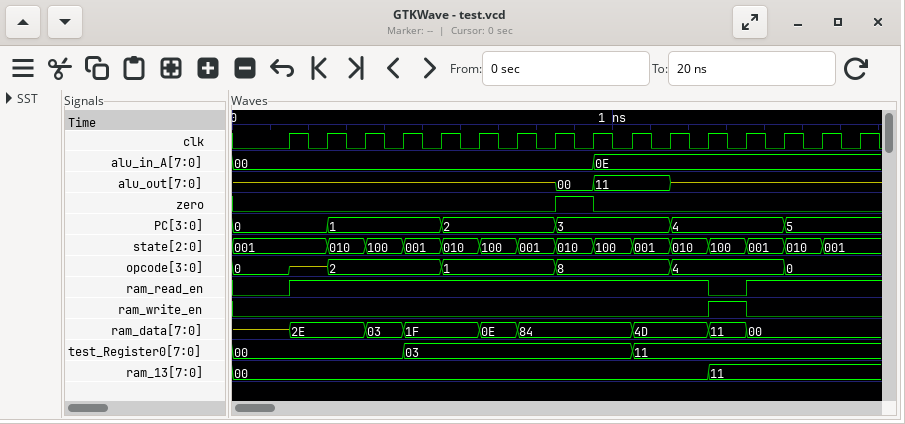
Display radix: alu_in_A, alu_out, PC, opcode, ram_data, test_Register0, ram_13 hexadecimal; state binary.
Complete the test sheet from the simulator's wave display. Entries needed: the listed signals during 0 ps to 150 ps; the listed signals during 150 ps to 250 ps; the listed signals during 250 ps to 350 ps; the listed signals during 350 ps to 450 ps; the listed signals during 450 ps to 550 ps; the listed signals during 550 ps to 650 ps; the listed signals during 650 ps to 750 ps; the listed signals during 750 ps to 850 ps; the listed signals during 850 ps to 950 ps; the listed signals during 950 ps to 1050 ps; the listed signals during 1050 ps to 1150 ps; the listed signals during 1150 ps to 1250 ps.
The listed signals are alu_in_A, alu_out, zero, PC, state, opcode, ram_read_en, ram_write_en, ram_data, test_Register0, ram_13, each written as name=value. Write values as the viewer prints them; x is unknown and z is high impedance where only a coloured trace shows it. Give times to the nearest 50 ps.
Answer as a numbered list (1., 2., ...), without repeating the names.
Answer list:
1. alu_in_A=00, alu_out=z, zero=0, PC=0, state=001, opcode=0, ram_read_en=0, ram_write_en=0, ram_data=z, test_Register0=00, ram_13=00
2. alu_in_A=00, alu_out=z, zero=0, PC=0, state=001, opcode=z, ram_read_en=1, ram_write_en=0, ram_data=2E, test_Register0=00, ram_13=00
3. alu_in_A=00, alu_out=z, zero=0, PC=1, state=010, opcode=2, ram_read_en=1, ram_write_en=0, ram_data=2E, test_Register0=00, ram_13=00
4. alu_in_A=00, alu_out=z, zero=0, PC=1, state=100, opcode=2, ram_read_en=1, ram_write_en=0, ram_data=03, test_Register0=00, ram_13=00
5. alu_in_A=00, alu_out=z, zero=0, PC=1, state=001, opcode=2, ram_read_en=1, ram_write_en=0, ram_data=1F, test_Register0=03, ram_13=00
6. alu_in_A=00, alu_out=z, zero=0, PC=2, state=010, opcode=1, ram_read_en=1, ram_write_en=0, ram_data=1F, test_Register0=03, ram_13=00
7. alu_in_A=00, alu_out=z, zero=0, PC=2, state=100, opcode=1, ram_read_en=1, ram_write_en=0, ram_data=0E, test_Register0=03, ram_13=00
8. alu_in_A=00, alu_out=z, zero=0, PC=2, state=001, opcode=1, ram_read_en=1, ram_write_en=0, ram_data=84, test_Register0=03, ram_13=00
9. alu_in_A=00, alu_out=00, zero=1, PC=3, state=010, opcode=8, ram_read_en=1, ram_write_en=0, ram_data=84, test_Register0=03, ram_13=00
10. alu_in_A=0E, alu_out=11, zero=0, PC=3, state=100, opcode=8, ram_read_en=1, ram_write_en=0, ram_data=84, test_Register0=03, ram_13=00
11. alu_in_A=0E, alu_out=11, zero=0, PC=3, state=001, opcode=8, ram_read_en=1, ram_write_en=0, ram_data=4D, test_Register0=11, ram_13=00
12. alu_in_A=0E, alu_out=z, zero=0, PC=4, state=010, opcode=4, ram_read_en=1, ram_write_en=0, ram_data=4D, test_Register0=11, ram_13=00
